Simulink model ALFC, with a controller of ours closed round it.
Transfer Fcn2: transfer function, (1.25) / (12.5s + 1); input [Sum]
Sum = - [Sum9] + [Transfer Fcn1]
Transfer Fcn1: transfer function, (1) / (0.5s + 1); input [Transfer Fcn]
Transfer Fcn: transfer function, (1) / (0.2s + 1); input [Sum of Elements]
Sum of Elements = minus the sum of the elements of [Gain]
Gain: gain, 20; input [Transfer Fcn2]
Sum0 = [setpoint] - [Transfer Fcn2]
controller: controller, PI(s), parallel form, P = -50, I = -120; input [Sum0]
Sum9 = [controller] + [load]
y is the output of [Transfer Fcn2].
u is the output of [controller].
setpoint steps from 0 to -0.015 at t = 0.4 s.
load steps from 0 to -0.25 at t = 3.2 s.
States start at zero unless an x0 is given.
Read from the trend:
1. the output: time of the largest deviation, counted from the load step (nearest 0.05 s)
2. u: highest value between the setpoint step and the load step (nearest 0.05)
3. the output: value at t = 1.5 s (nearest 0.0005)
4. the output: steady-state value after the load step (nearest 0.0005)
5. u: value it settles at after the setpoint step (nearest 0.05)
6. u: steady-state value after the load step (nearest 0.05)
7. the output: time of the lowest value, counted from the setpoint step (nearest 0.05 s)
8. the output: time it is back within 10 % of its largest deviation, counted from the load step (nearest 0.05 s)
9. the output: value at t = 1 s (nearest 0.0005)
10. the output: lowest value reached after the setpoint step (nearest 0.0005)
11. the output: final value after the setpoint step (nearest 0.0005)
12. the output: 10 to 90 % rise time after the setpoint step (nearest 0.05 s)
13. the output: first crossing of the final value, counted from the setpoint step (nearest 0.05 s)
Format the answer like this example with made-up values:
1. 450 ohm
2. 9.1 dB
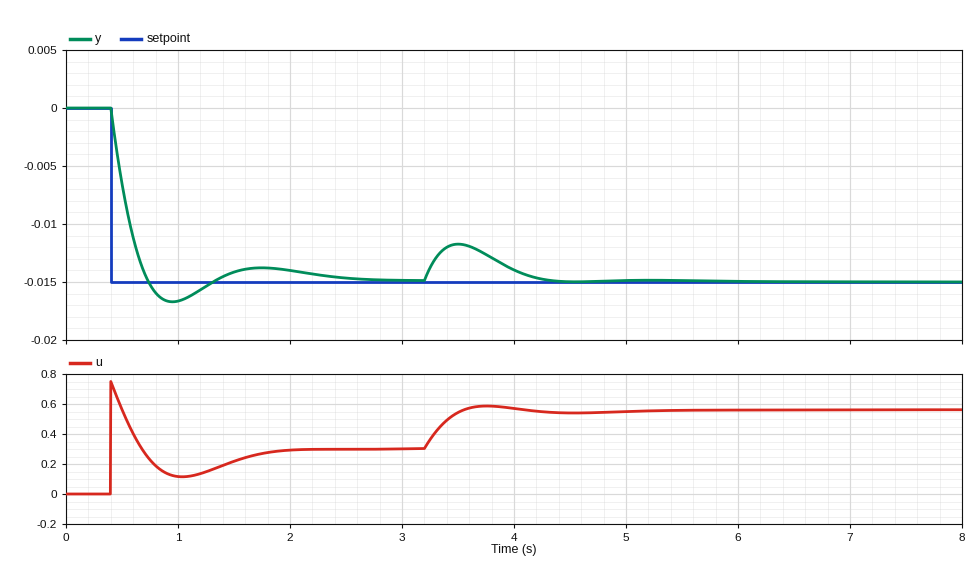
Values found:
1. 0.30 s
2. 0.75
3. -0.0140
4. -0.0150
5. 0.30
6. 0.55
7. 0.55 s
8. 1.00 s
9. -0.0165
10. -0.0165
11. -0.0150
12. 0.25 s
13. 0.35 s
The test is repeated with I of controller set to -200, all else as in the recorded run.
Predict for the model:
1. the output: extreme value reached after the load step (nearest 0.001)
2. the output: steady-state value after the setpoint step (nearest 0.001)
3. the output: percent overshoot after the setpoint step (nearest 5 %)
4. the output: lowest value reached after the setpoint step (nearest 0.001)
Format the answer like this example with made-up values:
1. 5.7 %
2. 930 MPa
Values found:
1. -0.012
2. -0.015
3. 20 %
4. -0.018
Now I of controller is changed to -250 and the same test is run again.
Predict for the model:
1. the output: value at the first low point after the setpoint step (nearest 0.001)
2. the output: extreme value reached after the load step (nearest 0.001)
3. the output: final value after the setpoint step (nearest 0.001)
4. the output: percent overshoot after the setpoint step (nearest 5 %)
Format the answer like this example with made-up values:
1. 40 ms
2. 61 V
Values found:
1. -0.019
2. -0.012
3. -0.015
4. 25 %
